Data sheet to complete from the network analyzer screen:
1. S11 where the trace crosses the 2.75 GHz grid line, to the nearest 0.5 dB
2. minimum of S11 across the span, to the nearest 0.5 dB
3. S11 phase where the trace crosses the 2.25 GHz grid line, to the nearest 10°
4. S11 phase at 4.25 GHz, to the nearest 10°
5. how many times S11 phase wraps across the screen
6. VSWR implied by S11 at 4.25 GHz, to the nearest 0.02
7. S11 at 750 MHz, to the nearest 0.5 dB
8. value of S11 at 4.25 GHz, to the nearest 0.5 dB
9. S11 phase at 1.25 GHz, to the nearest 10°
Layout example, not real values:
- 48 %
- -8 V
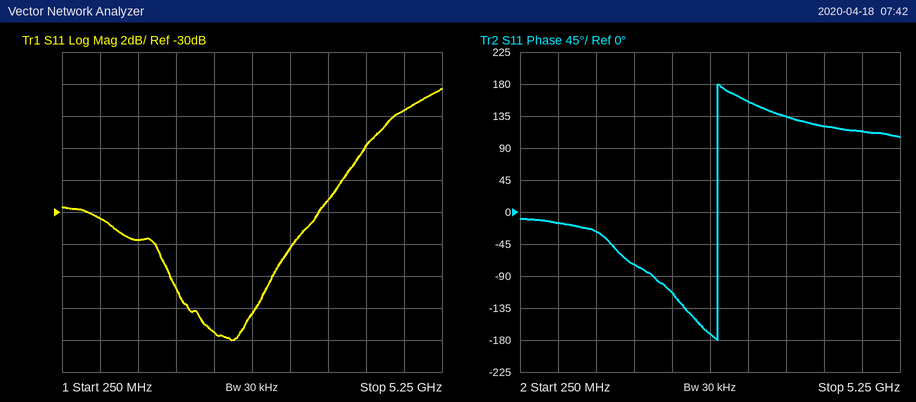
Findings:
- -36.5 dB
- -38.0 dB
- -110°
- 120°
- 1
- 1.10
- -30.5 dB
- -26.0 dB
- -30°
